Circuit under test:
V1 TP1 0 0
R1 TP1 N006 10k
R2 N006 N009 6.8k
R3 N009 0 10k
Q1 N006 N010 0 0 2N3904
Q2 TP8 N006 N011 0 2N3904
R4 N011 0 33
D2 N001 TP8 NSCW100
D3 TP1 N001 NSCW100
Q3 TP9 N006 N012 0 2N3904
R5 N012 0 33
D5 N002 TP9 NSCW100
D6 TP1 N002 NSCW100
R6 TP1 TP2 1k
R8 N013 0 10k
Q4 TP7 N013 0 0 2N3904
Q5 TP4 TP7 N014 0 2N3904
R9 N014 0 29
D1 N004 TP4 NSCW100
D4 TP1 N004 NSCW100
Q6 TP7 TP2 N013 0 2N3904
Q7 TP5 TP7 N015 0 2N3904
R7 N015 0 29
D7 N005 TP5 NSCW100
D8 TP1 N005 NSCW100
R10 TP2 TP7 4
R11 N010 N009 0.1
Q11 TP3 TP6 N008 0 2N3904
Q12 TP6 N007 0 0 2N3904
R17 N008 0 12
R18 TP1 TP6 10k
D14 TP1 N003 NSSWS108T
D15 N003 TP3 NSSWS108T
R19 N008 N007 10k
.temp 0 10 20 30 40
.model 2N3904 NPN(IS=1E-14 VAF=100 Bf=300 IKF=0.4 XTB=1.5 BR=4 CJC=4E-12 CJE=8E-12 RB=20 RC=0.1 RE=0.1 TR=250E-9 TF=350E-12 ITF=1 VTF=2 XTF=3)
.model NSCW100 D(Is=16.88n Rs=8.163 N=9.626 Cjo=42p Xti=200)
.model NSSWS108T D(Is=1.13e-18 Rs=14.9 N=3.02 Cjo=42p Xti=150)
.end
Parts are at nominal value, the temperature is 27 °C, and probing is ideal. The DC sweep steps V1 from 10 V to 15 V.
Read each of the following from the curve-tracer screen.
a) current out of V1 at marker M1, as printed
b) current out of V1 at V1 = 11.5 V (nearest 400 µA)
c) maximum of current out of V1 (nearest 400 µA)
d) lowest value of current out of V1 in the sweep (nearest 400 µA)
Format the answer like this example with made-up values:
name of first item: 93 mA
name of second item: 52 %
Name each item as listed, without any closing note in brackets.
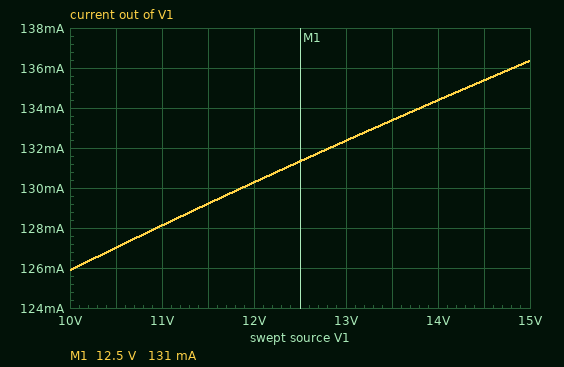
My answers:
current out of V1 at marker M1, as printed: 131 mA
current out of V1 at V1 = 11.5 V: 129.2 mA
maximum of current out of V1: 136.4 mA
lowest value of current out of V1 in the sweep: 126.0 mA
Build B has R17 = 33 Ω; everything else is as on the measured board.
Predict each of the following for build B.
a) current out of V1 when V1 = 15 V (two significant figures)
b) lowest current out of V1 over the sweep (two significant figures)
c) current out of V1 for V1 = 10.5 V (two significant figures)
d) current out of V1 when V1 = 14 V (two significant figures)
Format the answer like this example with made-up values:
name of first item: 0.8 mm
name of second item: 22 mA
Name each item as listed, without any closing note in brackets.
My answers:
current out of V1 when V1 = 15 V: 100 mA
lowest current out of V1 over the sweep: 91 mA
current out of V1 for V1 = 10.5 V: 92 mA
current out of V1 when V1 = 14 V: 98 mA
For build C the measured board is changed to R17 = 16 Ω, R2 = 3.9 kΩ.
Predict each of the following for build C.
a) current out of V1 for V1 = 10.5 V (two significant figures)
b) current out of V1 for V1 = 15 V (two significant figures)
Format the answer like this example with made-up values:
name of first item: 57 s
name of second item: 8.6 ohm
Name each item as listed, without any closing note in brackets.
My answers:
current out of V1 for V1 = 10.5 V: 100 mA
current out of V1 for V1 = 15 V: 110 mA
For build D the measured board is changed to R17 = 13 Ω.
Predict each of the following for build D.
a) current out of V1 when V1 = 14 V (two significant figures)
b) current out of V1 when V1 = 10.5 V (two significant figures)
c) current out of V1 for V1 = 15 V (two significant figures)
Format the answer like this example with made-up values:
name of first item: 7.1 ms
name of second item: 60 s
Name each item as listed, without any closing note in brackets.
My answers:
current out of V1 when V1 = 14 V: 130 mA
current out of V1 when V1 = 10.5 V: 120 mA
current out of V1 for V1 = 15 V: 130 mA
